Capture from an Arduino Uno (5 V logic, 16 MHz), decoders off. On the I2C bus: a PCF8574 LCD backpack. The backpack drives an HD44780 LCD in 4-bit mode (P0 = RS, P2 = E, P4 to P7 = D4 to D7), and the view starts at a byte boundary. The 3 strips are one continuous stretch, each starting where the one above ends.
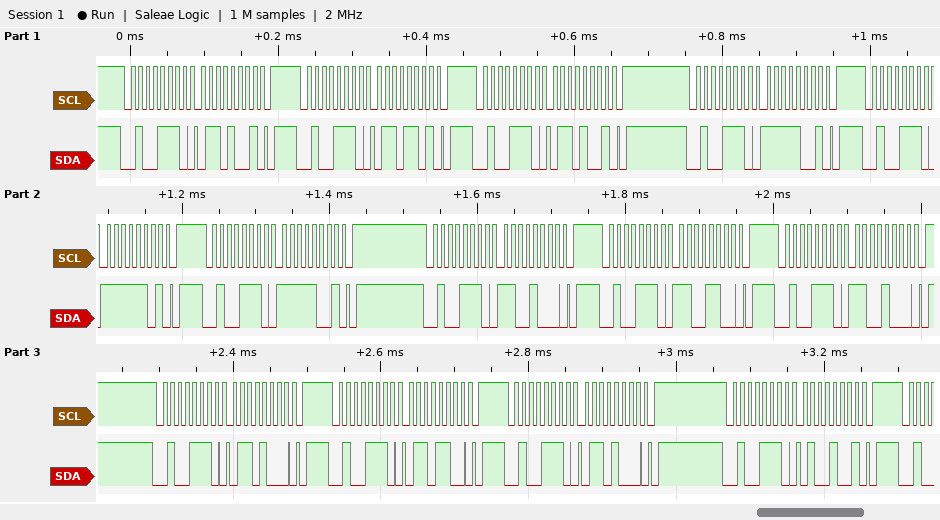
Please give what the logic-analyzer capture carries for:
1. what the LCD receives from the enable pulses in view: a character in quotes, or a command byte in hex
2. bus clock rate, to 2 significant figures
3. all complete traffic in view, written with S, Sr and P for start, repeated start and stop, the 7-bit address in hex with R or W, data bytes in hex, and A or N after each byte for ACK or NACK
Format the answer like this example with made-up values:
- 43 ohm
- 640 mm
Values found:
- 'o' 0xC6
- 100 kHz
- S 27W A 69 A P S 27W A 6D A P S 27W A 69 A P S 27W A F9 A P S 27W A FD A P S 27W A F9 A P S 27W A C8 A P S 27W A CC A P S 27W A C8 A P S 27W A 68 A P S 27W A 6C A P S 27W A 68 A P S 27W A 49 A P
